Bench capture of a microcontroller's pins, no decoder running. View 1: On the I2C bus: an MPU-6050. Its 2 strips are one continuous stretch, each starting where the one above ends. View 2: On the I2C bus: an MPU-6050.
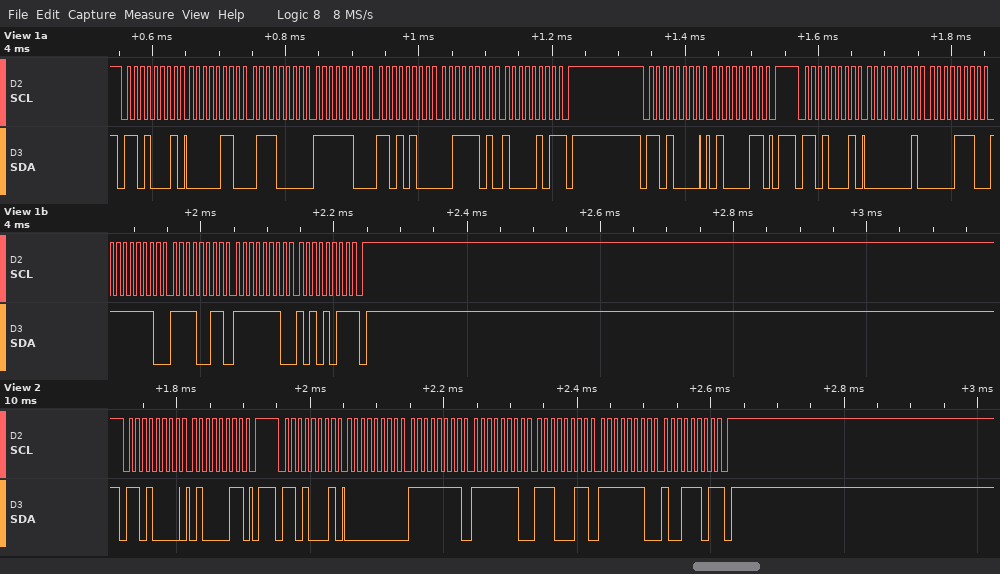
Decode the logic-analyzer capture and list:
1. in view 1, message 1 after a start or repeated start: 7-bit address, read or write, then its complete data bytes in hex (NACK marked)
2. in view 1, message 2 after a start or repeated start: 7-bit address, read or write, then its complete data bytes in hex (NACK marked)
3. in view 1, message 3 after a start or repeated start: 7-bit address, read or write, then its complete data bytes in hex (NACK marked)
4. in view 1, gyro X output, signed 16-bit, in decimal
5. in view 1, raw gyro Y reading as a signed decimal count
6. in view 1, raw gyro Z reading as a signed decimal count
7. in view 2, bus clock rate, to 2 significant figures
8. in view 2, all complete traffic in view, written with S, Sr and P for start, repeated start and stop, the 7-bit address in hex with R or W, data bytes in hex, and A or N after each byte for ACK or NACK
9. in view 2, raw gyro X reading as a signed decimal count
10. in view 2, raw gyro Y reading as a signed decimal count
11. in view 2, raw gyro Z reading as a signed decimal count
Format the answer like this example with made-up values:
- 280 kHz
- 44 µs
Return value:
- 0x68 read: 06 70 FC D4 3D 85 NACK
- 0x68 write: 43
- 0x68 read: 01 0E FE F3 FE AB NACK
- 270
- -269
- -341
- 100 kHz
- S 68W A 43 A P S 68R A 00 A FF A FE A E3 A FE A 9D N P
- 255
- -285
- -355
